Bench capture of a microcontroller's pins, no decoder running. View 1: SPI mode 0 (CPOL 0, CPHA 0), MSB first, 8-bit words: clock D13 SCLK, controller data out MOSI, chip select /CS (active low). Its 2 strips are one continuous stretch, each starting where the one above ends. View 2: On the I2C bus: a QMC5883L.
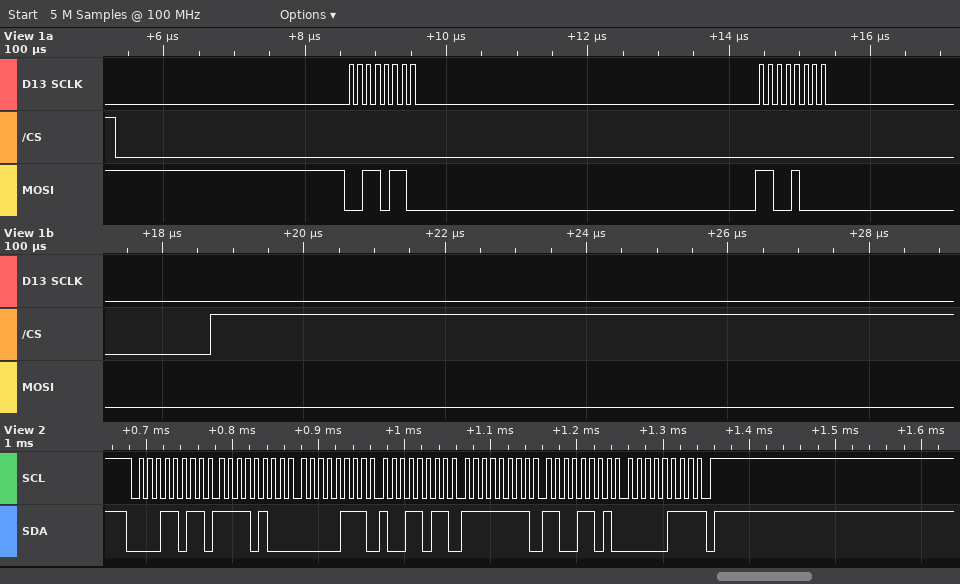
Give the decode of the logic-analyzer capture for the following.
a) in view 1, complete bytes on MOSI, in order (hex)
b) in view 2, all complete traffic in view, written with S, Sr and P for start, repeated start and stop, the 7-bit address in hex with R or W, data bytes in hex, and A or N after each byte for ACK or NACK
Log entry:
36 C8
S 0DR A F4 A 07 A 9B A FF A CD A 07 N P
